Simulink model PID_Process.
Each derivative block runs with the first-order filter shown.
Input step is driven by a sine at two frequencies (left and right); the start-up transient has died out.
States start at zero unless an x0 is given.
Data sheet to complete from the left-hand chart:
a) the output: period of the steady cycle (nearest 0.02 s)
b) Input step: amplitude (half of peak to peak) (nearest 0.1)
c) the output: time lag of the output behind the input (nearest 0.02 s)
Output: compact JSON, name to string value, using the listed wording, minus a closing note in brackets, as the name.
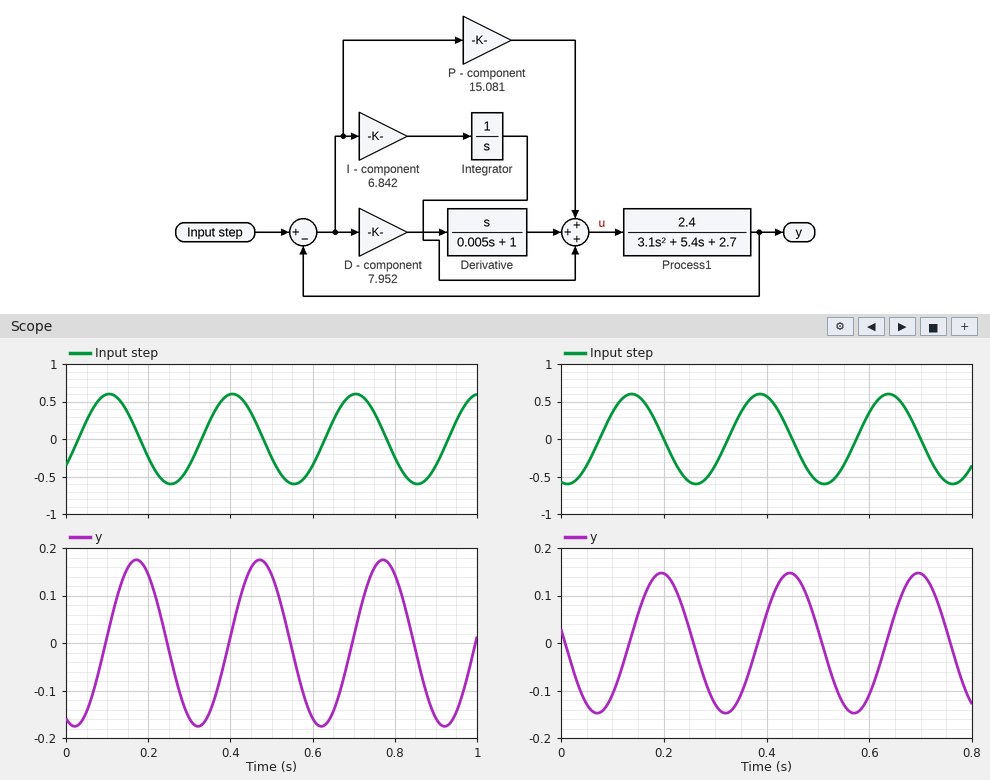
{"the output: period of the steady cycle": "0.30 s", "Input step: amplitude (half of peak to peak)": "0.6", "the output: time lag of the output behind the input": "0.06 s"}
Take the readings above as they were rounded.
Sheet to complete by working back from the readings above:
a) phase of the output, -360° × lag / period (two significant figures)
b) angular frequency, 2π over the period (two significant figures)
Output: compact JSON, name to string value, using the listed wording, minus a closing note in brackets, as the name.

{"phase of the output, -360° × lag / period": "-72°", "angular frequency, 2π over the period": "21 rad/s"}
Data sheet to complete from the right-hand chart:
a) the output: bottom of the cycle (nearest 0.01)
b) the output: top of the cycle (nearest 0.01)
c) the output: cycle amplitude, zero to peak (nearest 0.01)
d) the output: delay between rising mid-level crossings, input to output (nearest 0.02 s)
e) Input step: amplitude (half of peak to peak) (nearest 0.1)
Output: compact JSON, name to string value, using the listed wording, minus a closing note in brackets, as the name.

{"the output: bottom of the cycle": "-0.15", "the output: top of the cycle": "0.15", "the output: cycle amplitude, zero to peak": "0.15", "the output: delay between rising mid-level crossings, input to output": "0.06 s", "Input step: amplitude (half of peak to peak)": "0.6"}
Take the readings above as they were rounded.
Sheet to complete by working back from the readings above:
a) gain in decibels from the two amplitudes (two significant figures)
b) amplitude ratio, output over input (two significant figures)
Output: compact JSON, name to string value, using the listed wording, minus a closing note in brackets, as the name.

{"gain in decibels from the two amplitudes": "-12 dB", "amplitude ratio, output over input": "0.25"}
